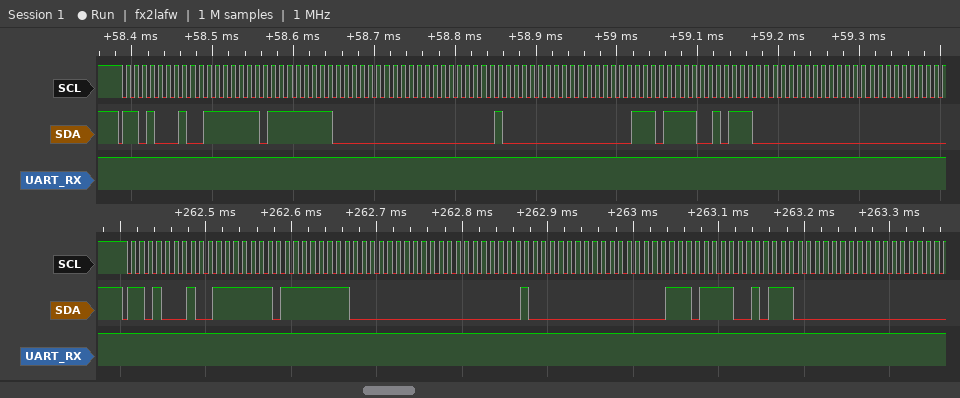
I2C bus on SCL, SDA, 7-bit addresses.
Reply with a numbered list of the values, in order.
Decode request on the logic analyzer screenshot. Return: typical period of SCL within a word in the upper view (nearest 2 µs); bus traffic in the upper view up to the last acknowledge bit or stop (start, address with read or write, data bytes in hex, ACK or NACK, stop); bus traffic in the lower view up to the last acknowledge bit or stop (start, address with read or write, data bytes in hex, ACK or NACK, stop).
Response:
1. 10 µs
2. start, address 68 read ACK, 7F ACK, FF ACK, 00 ACK, 00 ACK, 40 ACK, 00 ACK, EF ACK, 5C ACK, 00 ACK, 00 ACK
3. start, address 68 read ACK, 7F ACK, FF ACK, 00 ACK, 00 ACK, 40 ACK, 00 ACK, EF ACK, 5C ACK, 00 ACK
